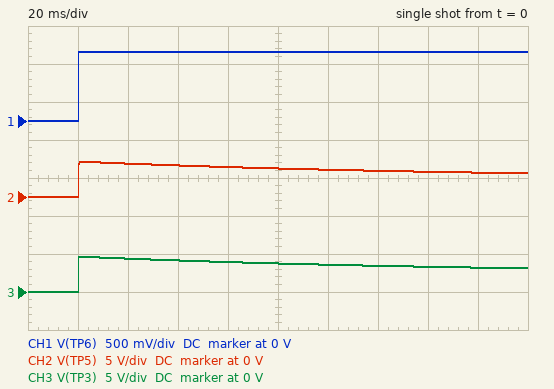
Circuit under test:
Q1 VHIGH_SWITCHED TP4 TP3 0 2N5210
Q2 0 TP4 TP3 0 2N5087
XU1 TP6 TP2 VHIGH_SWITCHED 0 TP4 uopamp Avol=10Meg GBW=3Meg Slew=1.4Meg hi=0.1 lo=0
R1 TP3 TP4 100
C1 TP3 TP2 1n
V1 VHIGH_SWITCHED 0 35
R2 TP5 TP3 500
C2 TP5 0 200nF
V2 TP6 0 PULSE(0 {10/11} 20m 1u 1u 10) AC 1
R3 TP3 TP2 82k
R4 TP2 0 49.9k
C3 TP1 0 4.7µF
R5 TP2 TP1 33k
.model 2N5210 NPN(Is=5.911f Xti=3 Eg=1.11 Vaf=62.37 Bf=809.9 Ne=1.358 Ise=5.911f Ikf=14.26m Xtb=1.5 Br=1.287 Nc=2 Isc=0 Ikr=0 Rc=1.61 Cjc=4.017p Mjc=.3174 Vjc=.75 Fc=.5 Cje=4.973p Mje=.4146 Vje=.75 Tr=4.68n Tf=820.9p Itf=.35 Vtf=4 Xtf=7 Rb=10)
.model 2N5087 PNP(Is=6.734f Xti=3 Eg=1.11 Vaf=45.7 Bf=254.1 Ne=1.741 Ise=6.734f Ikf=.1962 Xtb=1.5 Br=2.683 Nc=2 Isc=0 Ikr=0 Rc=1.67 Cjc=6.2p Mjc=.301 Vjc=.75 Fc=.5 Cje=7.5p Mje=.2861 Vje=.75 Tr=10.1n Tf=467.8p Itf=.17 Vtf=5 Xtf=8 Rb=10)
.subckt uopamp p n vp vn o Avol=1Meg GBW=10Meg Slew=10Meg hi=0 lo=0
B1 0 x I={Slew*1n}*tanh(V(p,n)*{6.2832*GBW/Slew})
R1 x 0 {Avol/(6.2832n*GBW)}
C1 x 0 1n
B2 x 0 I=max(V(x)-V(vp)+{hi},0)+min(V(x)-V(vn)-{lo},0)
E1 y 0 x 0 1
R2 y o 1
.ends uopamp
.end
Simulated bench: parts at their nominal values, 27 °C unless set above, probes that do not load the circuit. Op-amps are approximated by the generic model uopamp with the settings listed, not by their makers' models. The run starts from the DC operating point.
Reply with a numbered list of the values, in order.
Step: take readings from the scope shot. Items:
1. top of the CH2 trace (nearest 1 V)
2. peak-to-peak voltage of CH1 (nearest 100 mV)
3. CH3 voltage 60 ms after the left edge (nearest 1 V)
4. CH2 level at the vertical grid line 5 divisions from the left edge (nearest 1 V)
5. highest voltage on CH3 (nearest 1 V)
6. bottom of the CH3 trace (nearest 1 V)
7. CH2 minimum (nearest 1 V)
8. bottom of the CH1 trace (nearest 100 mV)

1. 5 V
2. 900 mV
3. 4 V
4. 4 V
5. 5 V
6. 0 V
7. 0 V
8. 0 V
